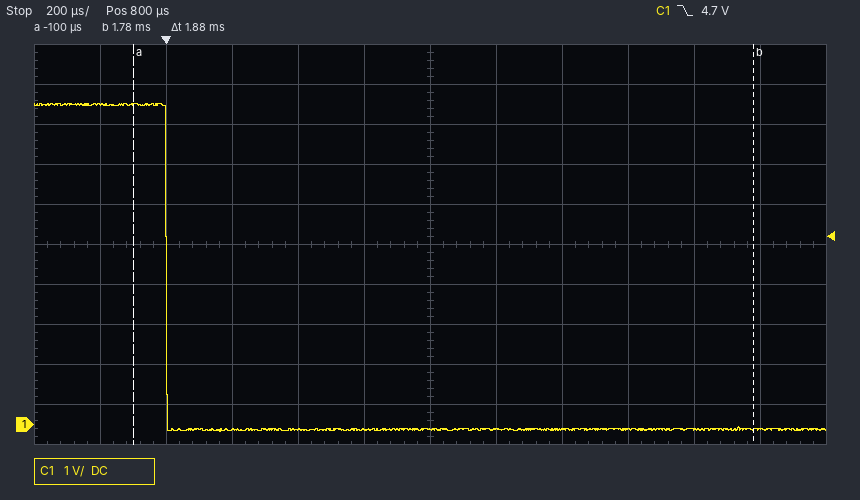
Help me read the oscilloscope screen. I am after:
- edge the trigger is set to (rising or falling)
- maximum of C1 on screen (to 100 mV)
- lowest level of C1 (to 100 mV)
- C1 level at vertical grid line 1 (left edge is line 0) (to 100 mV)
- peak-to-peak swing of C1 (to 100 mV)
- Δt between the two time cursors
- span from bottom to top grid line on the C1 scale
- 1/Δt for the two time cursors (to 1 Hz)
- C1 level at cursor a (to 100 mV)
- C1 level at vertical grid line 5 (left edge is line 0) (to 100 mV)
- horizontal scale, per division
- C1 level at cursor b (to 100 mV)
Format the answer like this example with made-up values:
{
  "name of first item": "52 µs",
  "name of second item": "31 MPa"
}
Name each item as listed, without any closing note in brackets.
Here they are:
{
  "edge the trigger is set to": "falling",
  "maximum of C1 on screen": "8.0 V",
  "lowest level of C1": "-200 mV",
  "C1 level at vertical grid line 1 (left edge is line 0)": "8.0 V",
  "peak-to-peak swing of C1": "8.2 V",
  "Δt between the two time cursors": "1.88 ms",
  "span from bottom to top grid line on the C1 scale": "10 V",
  "1/Δt for the two time cursors": "532 Hz",
  "C1 level at cursor a": "8.0 V",
  "C1 level at vertical grid line 5 (left edge is line 0)": "-100 mV",
  "horizontal scale, per division": "200 µs",
  "C1 level at cursor b": "-100 mV"
}
